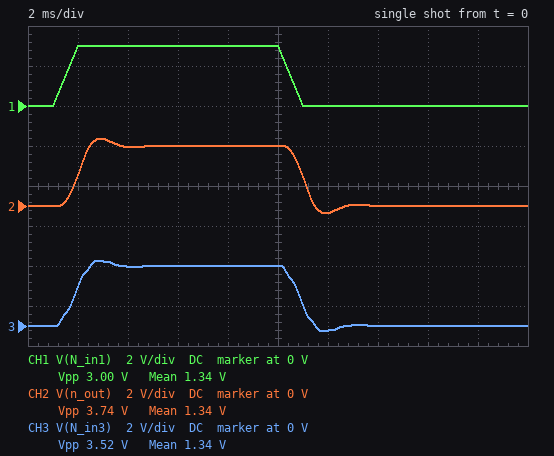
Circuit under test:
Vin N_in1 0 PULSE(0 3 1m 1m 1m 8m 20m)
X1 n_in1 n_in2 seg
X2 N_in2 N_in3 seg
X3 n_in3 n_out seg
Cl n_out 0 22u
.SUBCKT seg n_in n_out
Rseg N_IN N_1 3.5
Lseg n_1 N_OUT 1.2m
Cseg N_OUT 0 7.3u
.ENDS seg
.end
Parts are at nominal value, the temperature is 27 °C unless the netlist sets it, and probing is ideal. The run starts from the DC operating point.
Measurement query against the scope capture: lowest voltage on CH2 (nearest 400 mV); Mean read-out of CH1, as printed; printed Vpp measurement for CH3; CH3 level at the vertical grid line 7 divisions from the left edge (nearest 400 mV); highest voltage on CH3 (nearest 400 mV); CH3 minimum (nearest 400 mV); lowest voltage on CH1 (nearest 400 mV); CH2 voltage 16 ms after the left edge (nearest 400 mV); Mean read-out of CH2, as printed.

-400 mV
1.34 V
3.52 V
0 V
3.2 V
-400 mV
0 V
0 V
1.34 V
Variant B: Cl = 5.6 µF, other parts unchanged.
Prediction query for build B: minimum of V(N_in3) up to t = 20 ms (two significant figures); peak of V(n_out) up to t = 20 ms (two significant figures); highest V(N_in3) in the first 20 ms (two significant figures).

-390 mV
3.5 V
3.4 V
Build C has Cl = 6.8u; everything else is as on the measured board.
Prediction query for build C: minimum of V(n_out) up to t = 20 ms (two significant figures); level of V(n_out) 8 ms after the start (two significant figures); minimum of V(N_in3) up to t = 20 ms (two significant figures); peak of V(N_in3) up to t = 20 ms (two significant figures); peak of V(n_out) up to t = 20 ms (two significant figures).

-510 mV
3.0 V
-400 mV
3.4 V
3.5 V
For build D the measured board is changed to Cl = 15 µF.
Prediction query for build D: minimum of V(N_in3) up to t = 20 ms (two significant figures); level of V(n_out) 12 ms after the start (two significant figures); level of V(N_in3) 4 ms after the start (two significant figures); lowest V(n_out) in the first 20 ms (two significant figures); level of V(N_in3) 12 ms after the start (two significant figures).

-350 mV
-320 mV
2.9 V
-430 mV
-210 mV
